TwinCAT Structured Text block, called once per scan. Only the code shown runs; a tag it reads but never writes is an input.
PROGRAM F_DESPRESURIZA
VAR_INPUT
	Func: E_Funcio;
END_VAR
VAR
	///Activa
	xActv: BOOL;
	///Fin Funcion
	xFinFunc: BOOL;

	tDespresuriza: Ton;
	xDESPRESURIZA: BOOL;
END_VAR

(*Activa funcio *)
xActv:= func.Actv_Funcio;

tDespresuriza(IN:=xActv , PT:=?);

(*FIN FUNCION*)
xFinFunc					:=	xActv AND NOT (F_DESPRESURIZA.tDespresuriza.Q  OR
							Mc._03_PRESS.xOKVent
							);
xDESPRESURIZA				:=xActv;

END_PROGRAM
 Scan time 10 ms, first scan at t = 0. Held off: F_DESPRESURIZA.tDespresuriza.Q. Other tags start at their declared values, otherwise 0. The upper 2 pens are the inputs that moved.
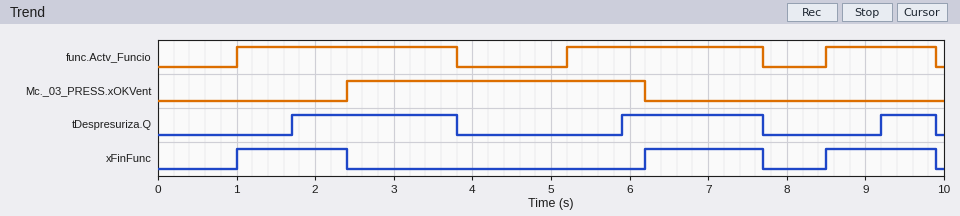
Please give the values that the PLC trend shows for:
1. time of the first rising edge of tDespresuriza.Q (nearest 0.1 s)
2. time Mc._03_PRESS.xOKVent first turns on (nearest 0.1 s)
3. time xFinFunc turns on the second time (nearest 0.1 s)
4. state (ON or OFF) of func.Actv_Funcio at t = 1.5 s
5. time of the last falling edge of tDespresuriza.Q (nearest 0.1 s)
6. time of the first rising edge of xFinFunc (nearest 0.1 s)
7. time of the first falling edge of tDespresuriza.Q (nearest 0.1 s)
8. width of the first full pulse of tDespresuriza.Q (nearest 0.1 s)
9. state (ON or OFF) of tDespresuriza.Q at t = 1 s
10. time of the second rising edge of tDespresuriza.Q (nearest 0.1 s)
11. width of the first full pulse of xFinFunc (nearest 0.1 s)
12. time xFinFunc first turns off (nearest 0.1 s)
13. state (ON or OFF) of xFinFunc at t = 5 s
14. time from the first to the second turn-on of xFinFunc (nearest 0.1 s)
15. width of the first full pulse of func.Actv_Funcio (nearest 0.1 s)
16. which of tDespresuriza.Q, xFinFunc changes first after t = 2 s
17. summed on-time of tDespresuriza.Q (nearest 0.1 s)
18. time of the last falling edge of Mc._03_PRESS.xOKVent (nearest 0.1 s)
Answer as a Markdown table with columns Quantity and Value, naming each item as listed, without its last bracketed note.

| Quantity | Value |
|---|---|
| time of the first rising edge of tDespresuriza.Q | 1.7 s |
| time Mc._03_PRESS.xOKVent first turns on | 2.4 s |
| time xFinFunc turns on the second time | 6.2 s |
| state (ON or OFF) of func.Actv_Funcio at t = 1.5 s | ON |
| time of the last falling edge of tDespresuriza.Q | 9.9 s |
| time of the first rising edge of xFinFunc | 1.0 s |
| time of the first falling edge of tDespresuriza.Q | 3.8 s |
| width of the first full pulse of tDespresuriza.Q | 2.1 s |
| state (ON or OFF) of tDespresuriza.Q at t = 1 s | OFF |
| time of the second rising edge of tDespresuriza.Q | 5.9 s |
| width of the first full pulse of xFinFunc | 1.4 s |
| time xFinFunc first turns off | 2.4 s |
| state (ON or OFF) of xFinFunc at t = 5 s | OFF |
| time from the first to the second turn-on of xFinFunc | 5.2 s |
| width of the first full pulse of func.Actv_Funcio | 2.8 s |
| which of tDespresuriza.Q, xFinFunc changes first after t = 2 s | xFinFunc |
| summed on-time of tDespresuriza.Q | 4.6 s |
| time of the last falling edge of Mc._03_PRESS.xOKVent | 6.2 s |
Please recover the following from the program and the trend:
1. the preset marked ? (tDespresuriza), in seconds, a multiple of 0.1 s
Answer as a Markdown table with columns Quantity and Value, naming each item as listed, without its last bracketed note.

| Quantity | Value |
|---|---|
| the preset marked ? (tDespresuriza), in seconds, a multiple of 0.1 s | 0.7 s |
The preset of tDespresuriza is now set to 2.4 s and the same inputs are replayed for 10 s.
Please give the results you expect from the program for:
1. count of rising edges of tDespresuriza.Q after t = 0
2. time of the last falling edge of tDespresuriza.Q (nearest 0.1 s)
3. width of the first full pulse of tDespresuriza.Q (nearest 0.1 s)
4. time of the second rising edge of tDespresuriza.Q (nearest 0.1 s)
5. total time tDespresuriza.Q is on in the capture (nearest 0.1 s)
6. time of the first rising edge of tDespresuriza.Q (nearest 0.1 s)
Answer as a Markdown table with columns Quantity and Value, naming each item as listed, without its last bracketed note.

| Quantity | Value |
|---|---|
| count of rising edges of tDespresuriza.Q after t = 0 | 2 |
| time of the last falling edge of tDespresuriza.Q | 7.7 s |
| width of the first full pulse of tDespresuriza.Q | 0.4 s |
| time of the second rising edge of tDespresuriza.Q | 7.6 s |
| total time tDespresuriza.Q is on in the capture | 0.5 s |
| time of the first rising edge of tDespresuriza.Q | 3.4 s |
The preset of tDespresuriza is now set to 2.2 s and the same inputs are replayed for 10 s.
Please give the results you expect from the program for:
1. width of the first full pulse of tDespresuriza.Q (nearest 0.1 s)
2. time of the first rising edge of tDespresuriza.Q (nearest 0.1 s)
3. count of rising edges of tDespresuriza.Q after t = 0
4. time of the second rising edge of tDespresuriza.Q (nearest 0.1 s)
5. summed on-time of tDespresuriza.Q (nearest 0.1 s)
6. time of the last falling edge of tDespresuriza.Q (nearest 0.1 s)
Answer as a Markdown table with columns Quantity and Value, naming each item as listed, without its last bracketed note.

| Quantity | Value |
|---|---|
| width of the first full pulse of tDespresuriza.Q | 0.6 s |
| time of the first rising edge of tDespresuriza.Q | 3.2 s |
| count of rising edges of tDespresuriza.Q after t = 0 | 2 |
| time of the second rising edge of tDespresuriza.Q | 7.4 s |
| summed on-time of tDespresuriza.Q | 0.9 s |
| time of the last falling edge of tDespresuriza.Q | 7.7 s |
